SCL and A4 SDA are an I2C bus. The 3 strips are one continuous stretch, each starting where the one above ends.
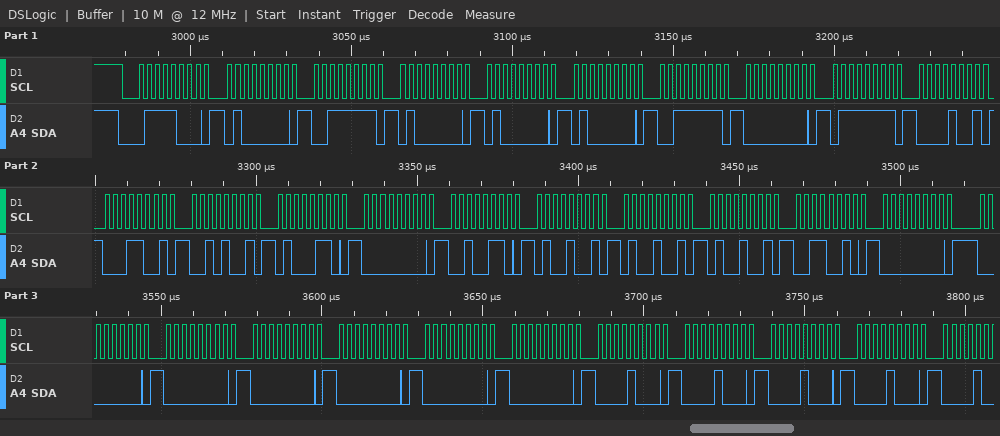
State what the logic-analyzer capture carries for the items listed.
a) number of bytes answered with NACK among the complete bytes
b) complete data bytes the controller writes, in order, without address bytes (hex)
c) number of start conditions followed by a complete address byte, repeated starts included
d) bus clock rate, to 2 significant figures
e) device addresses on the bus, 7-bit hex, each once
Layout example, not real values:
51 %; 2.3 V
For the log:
0; 40 3F 40 40 40 3F 00 7F 09 19 29 46 00 26 49 49 49 32 00 00 00 00 00 00 00 08 08 08 08; 1; 400 kHz; 0x3C
